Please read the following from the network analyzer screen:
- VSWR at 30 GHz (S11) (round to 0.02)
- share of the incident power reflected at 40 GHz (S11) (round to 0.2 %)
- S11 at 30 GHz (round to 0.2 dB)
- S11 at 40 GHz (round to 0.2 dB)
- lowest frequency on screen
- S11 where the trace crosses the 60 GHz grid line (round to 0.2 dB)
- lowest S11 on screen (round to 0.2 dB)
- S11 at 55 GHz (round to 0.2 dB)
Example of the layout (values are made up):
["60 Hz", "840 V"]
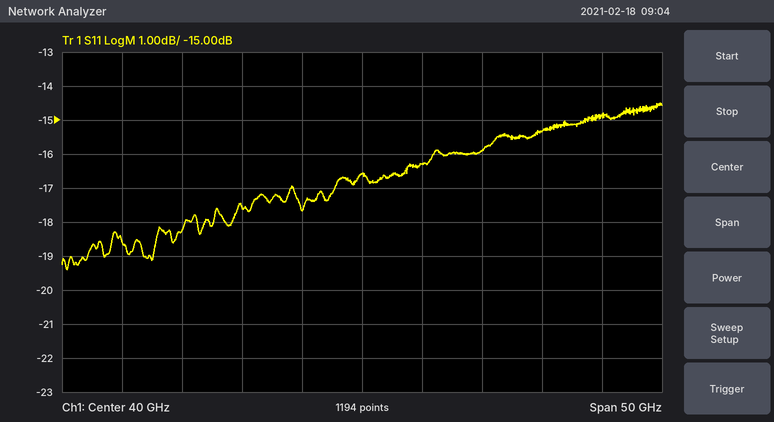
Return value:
["1.30", "2.2 %", "-17.6 dB", "-16.6 dB", "15 GHz", "-14.8 dB", "-19.4 dB", "-15.4 dB"]
